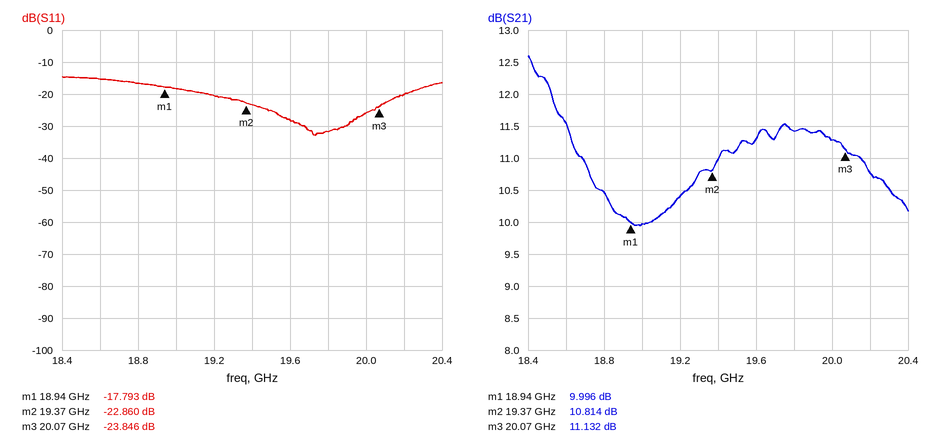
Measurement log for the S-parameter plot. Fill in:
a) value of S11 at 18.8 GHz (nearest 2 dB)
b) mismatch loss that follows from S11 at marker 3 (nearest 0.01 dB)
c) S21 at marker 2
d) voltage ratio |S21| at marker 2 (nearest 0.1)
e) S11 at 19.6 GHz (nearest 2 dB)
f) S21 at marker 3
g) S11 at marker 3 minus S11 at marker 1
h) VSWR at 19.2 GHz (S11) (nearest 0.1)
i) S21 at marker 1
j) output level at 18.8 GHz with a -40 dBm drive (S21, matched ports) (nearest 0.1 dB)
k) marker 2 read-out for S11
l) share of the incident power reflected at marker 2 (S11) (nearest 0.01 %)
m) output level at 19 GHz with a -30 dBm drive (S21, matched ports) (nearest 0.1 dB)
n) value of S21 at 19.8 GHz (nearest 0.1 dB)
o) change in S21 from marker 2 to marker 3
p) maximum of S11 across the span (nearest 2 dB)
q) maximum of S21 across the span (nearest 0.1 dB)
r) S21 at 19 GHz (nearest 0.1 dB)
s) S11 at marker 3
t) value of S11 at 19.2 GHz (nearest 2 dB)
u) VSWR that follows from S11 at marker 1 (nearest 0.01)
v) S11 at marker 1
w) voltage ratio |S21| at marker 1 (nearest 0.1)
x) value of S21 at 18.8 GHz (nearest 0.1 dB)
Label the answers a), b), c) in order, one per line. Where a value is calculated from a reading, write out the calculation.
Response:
a) -16 dB
b) −10 log10(1 − 10^(-23.846/10)) ≈ 0.02 dB
c) 10.814 dB
d) 10^(10.814/20) ≈ 3.5
e) -28 dB
f) 11.132 dB
g) -23.846 − (-17.793) = -6.053 dB
h) |Γ| = 10^(-20/20) = 0.1000; VSWR = (1 + 0.1000)/(1 − 0.1000) ≈ 1.2
i) 9.996 dB
j) -40 dBm + (10.5 dB) = -29.5 dBm
k) -22.860 dB
l) 10^(-22.86/10) ≈ 0.52 %
m) -30 dBm + (10.0 dB) = -20.0 dBm
n) 11.4 dB
o) 11.132 − (10.814) = 0.318 dB
p) -14 dB
q) 12.6 dB
r) 10.0 dB
s) -23.846 dB
t) -20 dB
u) (1 + 0.1289)/(1 − 0.1289) ≈ 1.30
v) -17.793 dB
w) 10^(9.996/20) ≈ 3.2
x) 10.5 dB
